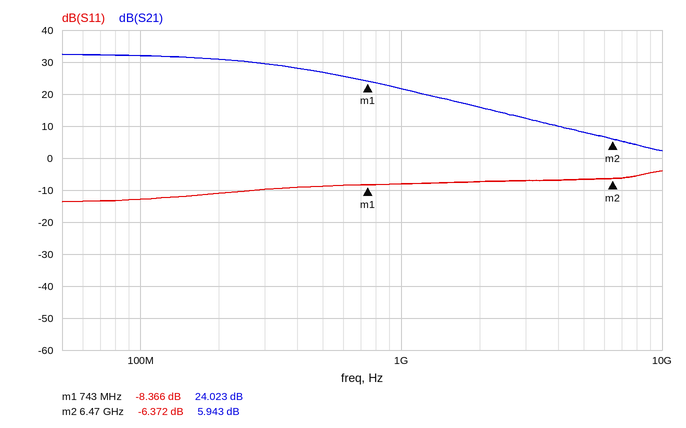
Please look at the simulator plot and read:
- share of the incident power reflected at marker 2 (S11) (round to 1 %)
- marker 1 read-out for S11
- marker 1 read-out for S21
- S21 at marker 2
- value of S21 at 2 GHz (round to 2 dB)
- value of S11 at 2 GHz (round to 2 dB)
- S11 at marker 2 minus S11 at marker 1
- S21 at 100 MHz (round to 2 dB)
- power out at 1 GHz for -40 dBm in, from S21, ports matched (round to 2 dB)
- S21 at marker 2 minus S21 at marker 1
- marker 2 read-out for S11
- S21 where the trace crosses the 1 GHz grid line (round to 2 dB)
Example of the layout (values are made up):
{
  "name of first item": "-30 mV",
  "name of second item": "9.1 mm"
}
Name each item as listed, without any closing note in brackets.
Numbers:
{
  "share of the incident power reflected at marker 2 (S11)": "23 %",
  "marker 1 read-out for S11": "-8.366 dB",
  "marker 1 read-out for S21": "24.023 dB",
  "S21 at marker 2": "5.943 dB",
  "value of S21 at 2 GHz": "16 dB",
  "value of S11 at 2 GHz": "-8 dB",
  "S11 at marker 2 minus S11 at marker 1": "1.994 dB",
  "S21 at 100 MHz": "32 dB",
  "power out at 1 GHz for -40 dBm in, from S21, ports matched": "-18 dBm",
  "S21 at marker 2 minus S21 at marker 1": "-18.080 dB",
  "marker 2 read-out for S11": "-6.372 dB",
  "S21 where the trace crosses the 1 GHz grid line": "22 dB"
}
